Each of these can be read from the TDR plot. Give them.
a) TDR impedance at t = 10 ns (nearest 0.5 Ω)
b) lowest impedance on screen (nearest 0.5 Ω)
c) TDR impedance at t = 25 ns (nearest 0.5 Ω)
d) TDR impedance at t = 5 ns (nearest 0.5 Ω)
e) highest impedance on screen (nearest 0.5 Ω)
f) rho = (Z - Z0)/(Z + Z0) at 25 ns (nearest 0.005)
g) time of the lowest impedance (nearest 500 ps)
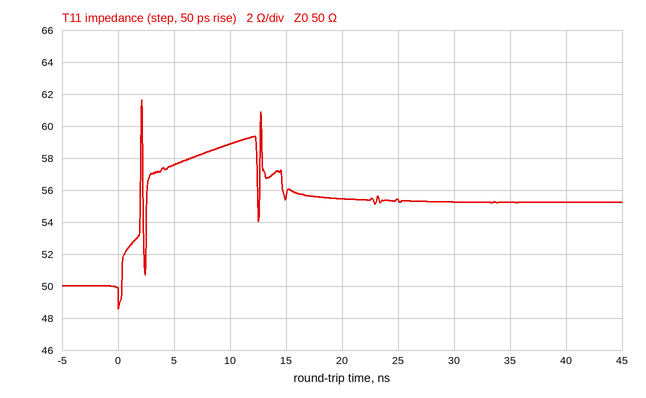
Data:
59.0 Ω
48.5 Ω
55.5 Ω
57.5 Ω
61.5 Ω
+0.050
0.0 ns
